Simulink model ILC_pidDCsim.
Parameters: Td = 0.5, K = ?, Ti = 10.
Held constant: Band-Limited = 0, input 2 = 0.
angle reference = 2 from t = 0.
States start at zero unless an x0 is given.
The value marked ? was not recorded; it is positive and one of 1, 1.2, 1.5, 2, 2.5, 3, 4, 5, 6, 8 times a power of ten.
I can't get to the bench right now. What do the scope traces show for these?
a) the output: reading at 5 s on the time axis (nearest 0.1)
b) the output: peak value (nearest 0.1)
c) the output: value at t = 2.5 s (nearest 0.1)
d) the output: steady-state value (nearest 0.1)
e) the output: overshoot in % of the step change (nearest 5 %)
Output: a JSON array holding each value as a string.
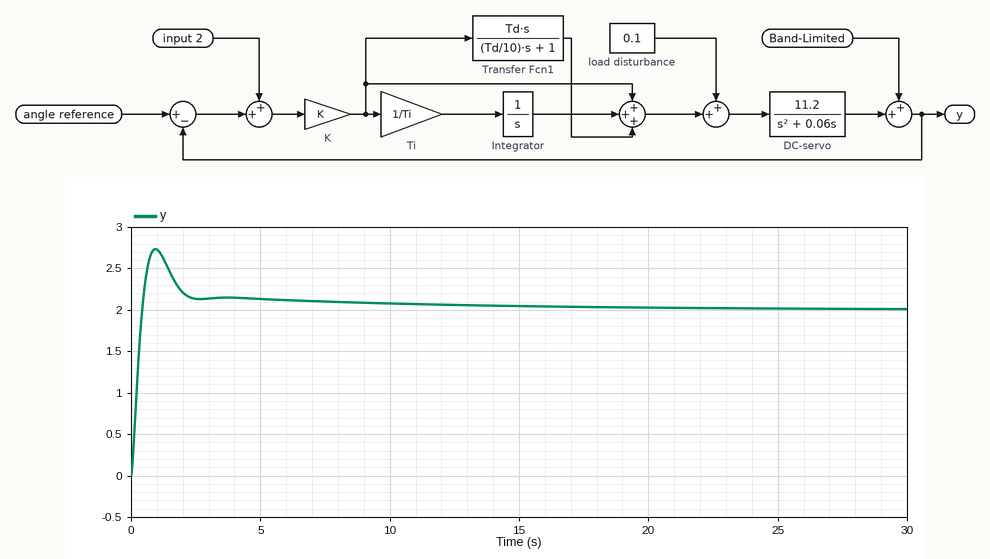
["2.1", "2.7", "2.1", "2.0", "35 %"]
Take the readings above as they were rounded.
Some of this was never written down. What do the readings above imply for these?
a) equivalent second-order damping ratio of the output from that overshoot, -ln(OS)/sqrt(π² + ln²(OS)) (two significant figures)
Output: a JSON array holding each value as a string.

["0.32"]
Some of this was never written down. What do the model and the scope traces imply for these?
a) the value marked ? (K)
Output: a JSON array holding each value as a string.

["0.5"]
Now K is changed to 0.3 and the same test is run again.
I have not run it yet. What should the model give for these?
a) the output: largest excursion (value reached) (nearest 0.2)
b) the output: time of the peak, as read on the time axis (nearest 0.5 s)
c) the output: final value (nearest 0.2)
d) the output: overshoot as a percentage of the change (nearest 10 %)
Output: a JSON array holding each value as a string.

["3.0", "1.5 s", "2.0", "50 %"]
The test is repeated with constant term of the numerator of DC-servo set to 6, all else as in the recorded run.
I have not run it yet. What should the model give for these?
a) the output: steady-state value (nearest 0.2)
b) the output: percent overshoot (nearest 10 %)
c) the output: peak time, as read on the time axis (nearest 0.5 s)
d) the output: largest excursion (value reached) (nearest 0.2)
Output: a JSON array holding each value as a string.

["2.0", "50 %", "1.5 s", "3.0"]
